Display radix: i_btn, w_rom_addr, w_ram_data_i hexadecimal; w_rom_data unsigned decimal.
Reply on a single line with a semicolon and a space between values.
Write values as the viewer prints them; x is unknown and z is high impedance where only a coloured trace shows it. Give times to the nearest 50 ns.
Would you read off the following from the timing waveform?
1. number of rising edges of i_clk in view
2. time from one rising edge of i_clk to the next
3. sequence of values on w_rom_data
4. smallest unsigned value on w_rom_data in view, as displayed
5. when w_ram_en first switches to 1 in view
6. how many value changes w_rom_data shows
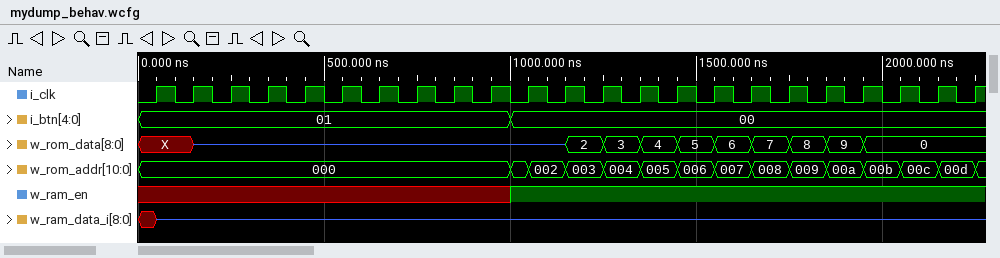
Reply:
23; 100 ns; X, z, 2, 3, 4, 5, 6, 7, 8, 9, 0; 0; 1000 ns; 10
